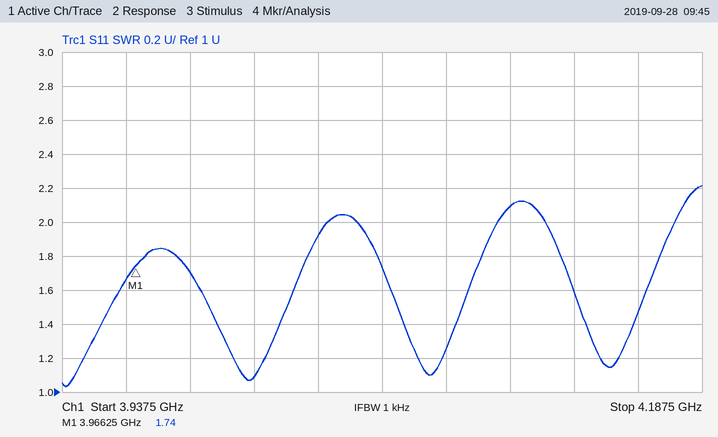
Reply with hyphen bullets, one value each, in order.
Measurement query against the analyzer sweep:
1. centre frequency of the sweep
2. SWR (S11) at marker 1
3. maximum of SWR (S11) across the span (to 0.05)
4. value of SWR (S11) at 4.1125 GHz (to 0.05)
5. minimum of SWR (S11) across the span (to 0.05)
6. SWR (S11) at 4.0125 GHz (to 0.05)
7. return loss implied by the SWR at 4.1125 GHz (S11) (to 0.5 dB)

- 4.0625 GHz
- 1.74
- 2.20
- 2.10
- 1.05
- 1.10
- 9.0 dB
